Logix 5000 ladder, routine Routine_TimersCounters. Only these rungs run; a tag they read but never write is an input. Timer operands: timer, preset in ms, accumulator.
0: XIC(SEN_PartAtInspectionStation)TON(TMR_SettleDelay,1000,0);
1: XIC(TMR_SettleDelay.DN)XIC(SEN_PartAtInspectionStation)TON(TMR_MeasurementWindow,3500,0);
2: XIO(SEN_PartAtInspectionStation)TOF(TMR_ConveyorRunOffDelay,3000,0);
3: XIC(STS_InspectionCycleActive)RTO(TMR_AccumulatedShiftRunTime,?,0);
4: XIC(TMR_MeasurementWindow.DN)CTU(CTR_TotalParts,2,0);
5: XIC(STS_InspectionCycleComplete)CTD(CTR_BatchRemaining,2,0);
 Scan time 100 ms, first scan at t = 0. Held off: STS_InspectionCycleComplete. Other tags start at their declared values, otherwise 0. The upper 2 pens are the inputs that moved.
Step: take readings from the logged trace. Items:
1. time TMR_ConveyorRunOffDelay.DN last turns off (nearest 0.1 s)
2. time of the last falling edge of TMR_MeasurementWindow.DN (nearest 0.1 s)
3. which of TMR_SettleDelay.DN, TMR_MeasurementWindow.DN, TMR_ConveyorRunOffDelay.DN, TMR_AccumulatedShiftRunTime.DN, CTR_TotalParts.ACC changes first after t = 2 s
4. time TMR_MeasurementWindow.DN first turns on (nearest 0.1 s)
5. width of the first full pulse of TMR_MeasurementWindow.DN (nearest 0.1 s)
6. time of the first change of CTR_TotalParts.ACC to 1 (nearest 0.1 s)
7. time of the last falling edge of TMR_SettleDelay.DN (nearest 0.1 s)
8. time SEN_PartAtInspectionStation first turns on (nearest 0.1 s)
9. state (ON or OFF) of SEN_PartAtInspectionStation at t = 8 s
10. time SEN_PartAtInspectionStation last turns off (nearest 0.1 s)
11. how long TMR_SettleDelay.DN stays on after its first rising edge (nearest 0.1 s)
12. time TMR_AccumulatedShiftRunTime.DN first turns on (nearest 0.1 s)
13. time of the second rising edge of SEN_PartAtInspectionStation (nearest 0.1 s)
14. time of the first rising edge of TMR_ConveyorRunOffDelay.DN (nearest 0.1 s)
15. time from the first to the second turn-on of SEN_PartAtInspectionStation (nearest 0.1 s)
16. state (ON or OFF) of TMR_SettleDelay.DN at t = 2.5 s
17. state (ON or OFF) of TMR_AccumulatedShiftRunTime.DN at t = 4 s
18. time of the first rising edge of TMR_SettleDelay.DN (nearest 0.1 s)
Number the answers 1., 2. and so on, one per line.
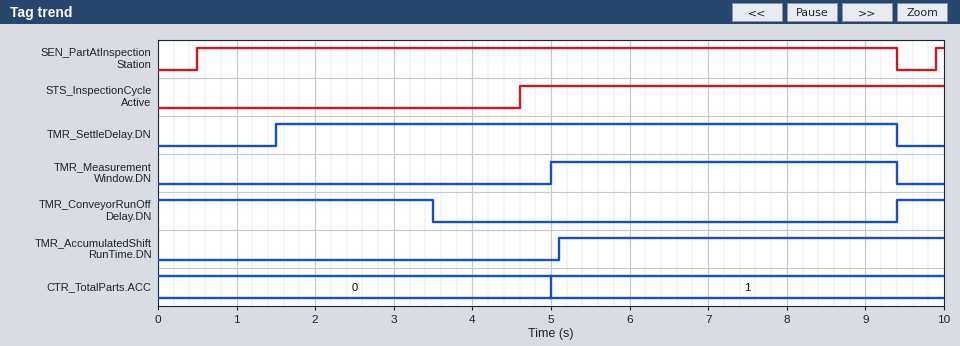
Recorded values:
1. 3.5 s
2. 9.4 s
3. TMR_ConveyorRunOffDelay.DN
4. 5.0 s
5. 4.4 s
6. 5.0 s
7. 9.4 s
8. 0.5 s
9. ON
10. 9.4 s
11. 7.9 s
12. 5.1 s
13. 9.9 s
14. 9.4 s
15. 9.4 s
16. ON
17. OFF
18. 1.5 s
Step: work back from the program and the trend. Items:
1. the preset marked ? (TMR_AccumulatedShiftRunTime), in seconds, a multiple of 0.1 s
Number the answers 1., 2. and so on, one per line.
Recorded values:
1. 0.5 s
